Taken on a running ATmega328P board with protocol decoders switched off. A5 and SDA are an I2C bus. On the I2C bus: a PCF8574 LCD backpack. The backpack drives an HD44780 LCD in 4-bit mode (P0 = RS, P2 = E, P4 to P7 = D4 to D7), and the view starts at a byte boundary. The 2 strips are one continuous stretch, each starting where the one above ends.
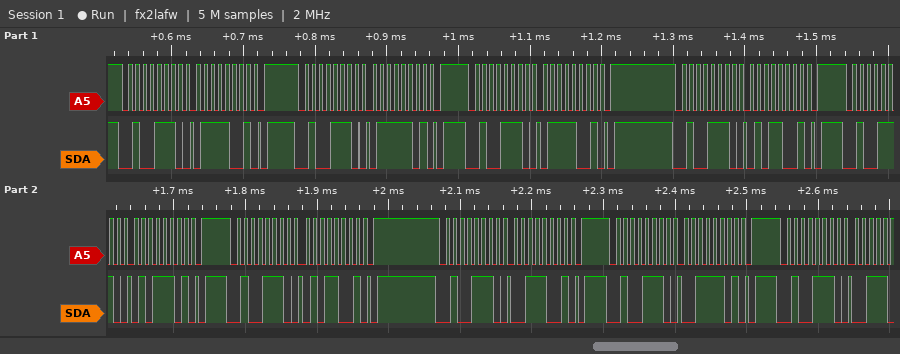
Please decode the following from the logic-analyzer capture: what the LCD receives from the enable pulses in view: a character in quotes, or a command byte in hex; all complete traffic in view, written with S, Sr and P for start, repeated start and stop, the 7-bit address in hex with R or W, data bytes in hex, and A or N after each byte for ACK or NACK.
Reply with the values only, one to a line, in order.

'u'
S 27W A 79 A P S 27W A 7D A P S 27W A 79 A P S 27W A 59 A P S 27W A 5D A P S 27W A 59 A P S 27W A 39 A P S 27W A 3D A P S 27W A
